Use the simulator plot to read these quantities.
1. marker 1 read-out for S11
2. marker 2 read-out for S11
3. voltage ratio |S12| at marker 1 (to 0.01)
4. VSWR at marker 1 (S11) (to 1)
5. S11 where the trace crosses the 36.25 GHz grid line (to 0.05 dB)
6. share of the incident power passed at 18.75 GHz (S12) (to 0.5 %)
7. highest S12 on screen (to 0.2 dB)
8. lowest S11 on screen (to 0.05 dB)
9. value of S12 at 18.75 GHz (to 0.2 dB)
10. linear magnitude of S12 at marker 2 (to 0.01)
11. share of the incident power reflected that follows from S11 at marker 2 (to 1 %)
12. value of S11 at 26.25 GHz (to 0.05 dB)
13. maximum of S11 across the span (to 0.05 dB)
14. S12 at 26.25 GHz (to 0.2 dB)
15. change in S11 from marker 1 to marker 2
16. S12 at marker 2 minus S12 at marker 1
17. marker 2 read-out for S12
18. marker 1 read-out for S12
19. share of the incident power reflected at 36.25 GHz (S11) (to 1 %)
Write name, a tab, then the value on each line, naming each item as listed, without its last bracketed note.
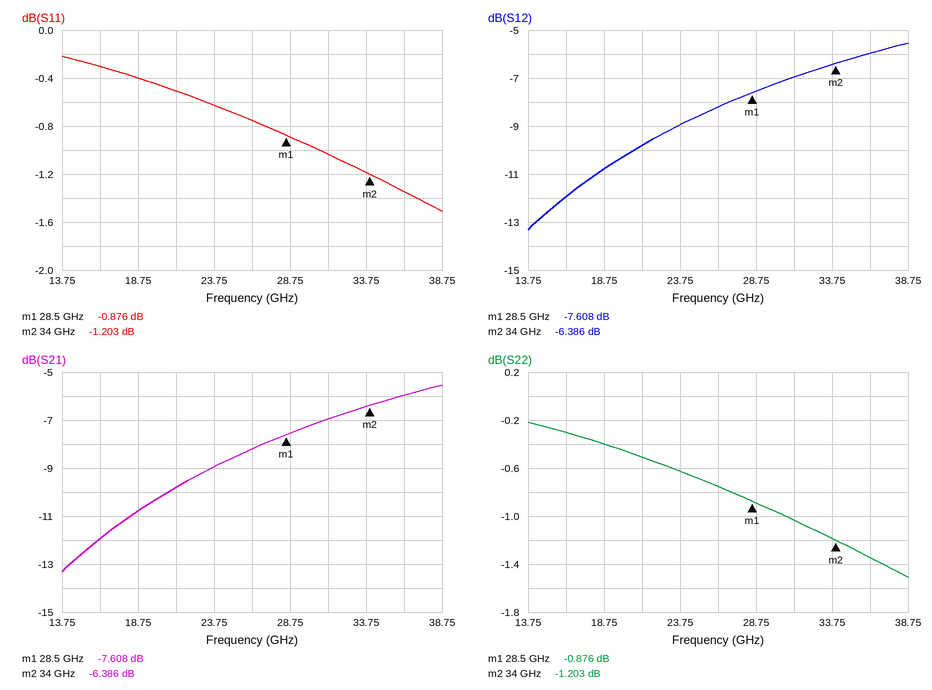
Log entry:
marker 1 read-out for S11	-0.876 dB
marker 2 read-out for S11	-1.203 dB
voltage ratio |S12| at marker 1	0.42
VSWR at marker 1 (S11)	20
S11 where the trace crosses the 36.25 GHz grid line	-1.35 dB
share of the incident power passed at 18.75 GHz (S12)	8.5 %
highest S12 on screen	-5.6 dB
lowest S11 on screen	-1.50 dB
value of S12 at 18.75 GHz	-10.8 dB
linear magnitude of S12 at marker 2	0.48
share of the incident power reflected that follows from S11 at marker 2	76 %
value of S11 at 26.25 GHz	-0.75 dB
maximum of S11 across the span	-0.20 dB
S12 at 26.25 GHz	-8.2 dB
change in S11 from marker 1 to marker 2	-0.327 dB
S12 at marker 2 minus S12 at marker 1	1.222 dB
marker 2 read-out for S12	-6.386 dB
marker 1 read-out for S12	-7.608 dB
share of the incident power reflected at 36.25 GHz (S11)	73 %
